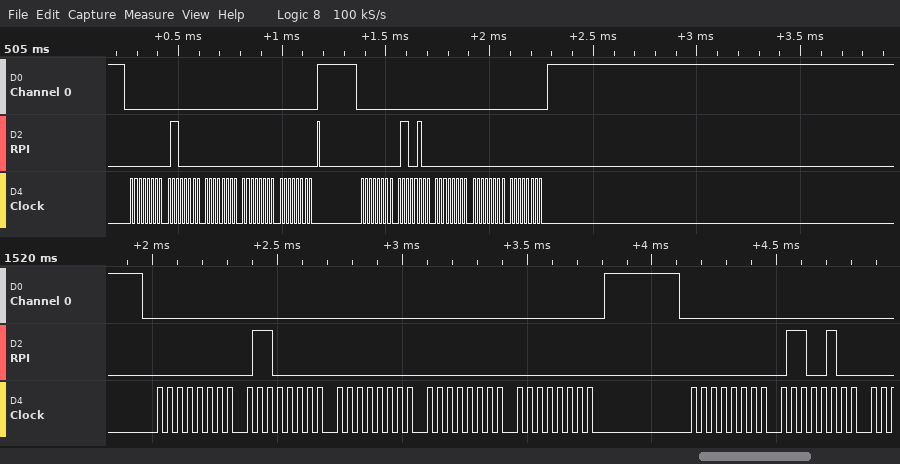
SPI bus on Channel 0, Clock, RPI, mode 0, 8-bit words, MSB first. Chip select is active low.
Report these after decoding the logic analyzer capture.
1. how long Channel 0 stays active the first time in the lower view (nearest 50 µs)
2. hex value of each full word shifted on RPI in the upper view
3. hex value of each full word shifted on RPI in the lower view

1850 µs
00, 60, 00, 00, 00, 00, 64, 00, 00, 00
00, 60, 00, 00, 00, 00, 64
